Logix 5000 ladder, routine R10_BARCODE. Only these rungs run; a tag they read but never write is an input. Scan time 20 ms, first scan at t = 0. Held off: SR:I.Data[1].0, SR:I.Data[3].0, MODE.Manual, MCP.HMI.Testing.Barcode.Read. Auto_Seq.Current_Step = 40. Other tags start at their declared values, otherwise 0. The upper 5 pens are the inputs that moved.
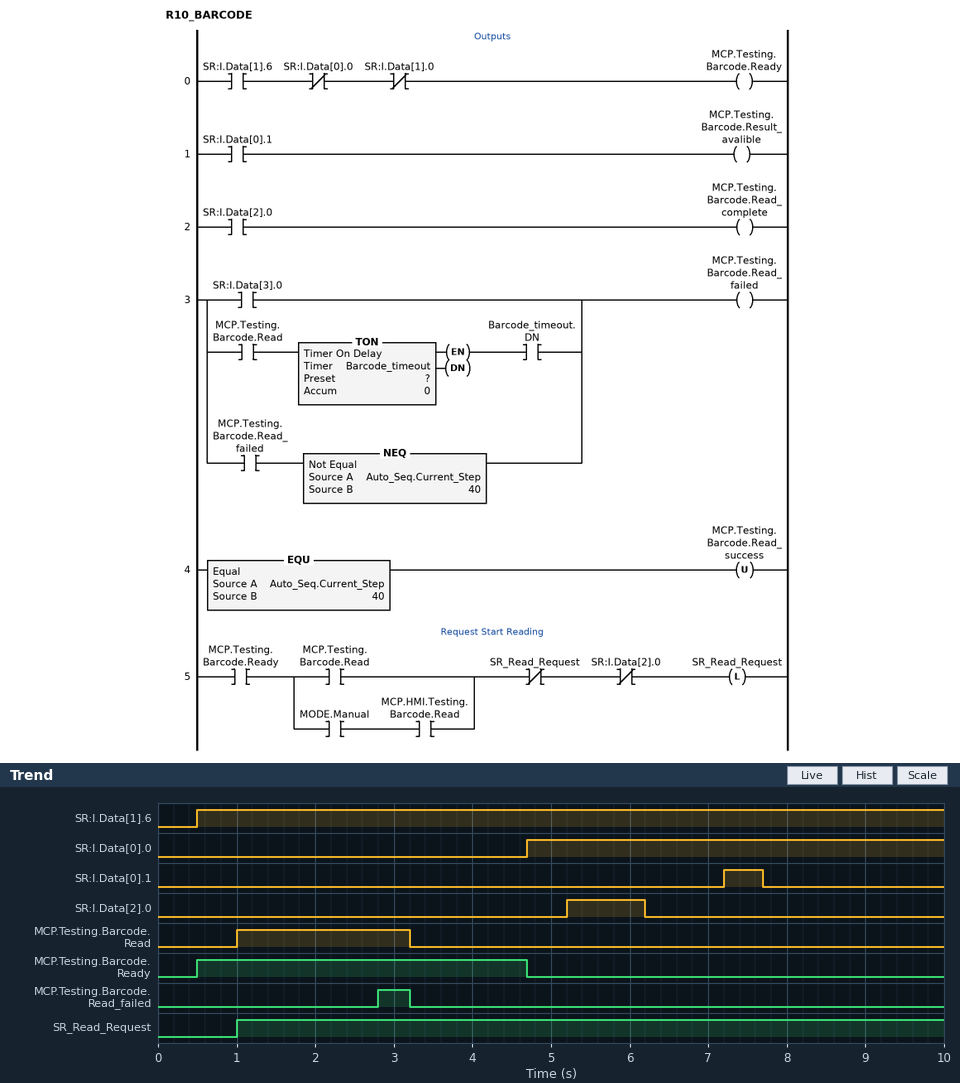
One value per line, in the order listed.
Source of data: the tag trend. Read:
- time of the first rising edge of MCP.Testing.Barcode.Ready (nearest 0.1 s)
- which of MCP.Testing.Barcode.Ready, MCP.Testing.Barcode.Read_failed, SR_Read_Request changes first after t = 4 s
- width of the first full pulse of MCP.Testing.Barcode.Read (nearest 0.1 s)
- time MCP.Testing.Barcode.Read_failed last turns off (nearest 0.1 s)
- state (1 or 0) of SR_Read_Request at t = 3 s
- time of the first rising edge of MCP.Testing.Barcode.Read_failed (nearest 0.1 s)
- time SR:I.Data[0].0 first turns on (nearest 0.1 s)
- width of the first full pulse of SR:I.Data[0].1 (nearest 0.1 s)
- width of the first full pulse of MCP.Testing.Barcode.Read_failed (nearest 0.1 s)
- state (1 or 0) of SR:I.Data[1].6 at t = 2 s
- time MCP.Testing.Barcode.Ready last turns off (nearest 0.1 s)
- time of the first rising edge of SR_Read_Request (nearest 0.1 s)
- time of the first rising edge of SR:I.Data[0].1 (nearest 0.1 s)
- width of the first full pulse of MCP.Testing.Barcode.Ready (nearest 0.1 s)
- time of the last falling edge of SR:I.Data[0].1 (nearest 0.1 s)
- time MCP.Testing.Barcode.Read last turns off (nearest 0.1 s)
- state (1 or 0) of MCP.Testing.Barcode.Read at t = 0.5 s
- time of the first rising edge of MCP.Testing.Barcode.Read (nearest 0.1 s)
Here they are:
0.5 s
MCP.Testing.Barcode.Ready
2.2 s
3.2 s
1
2.8 s
4.7 s
0.5 s
0.4 s
1
4.7 s
1.0 s
7.2 s
4.2 s
7.7 s
3.2 s
0
1.0 s
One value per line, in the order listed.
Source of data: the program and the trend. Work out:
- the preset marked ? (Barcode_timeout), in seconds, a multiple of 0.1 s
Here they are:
1.8 s
